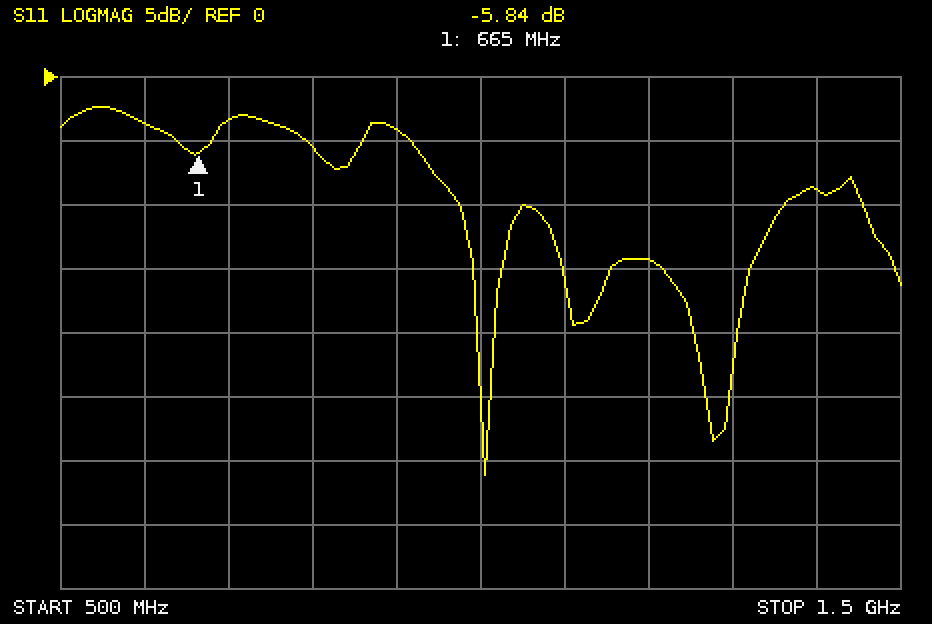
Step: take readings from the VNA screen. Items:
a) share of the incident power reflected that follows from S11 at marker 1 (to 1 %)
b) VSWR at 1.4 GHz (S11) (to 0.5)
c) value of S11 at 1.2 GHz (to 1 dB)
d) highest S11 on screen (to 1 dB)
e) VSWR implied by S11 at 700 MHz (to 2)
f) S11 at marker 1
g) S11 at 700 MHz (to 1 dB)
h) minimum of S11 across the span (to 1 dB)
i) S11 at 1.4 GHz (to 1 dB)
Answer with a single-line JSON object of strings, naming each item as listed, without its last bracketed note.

{"share of the incident power reflected that follows from S11 at marker 1": "26 %", "VSWR at 1.4 GHz (S11)": "2.0", "value of S11 at 1.2 GHz": "-14 dB", "highest S11 on screen": "-2 dB", "VSWR implied by S11 at 700 MHz": "6", "S11 at marker 1": "-5.84 dB", "S11 at 700 MHz": "-3 dB", "minimum of S11 across the span": "-31 dB", "S11 at 1.4 GHz": "-9 dB"}
